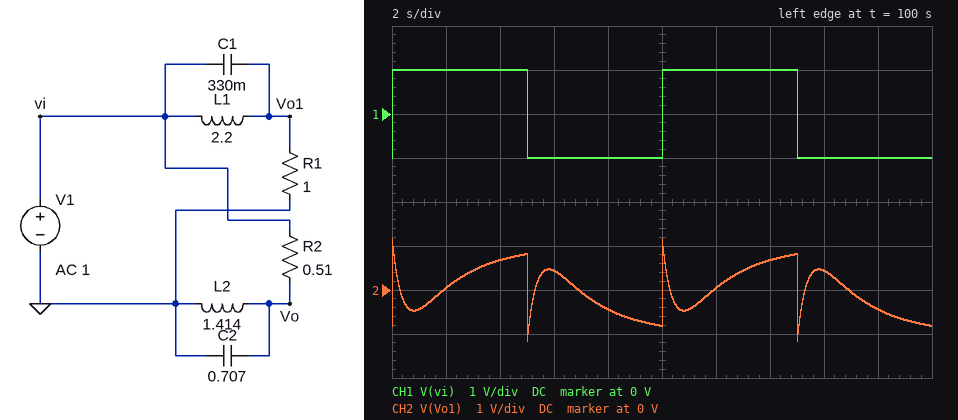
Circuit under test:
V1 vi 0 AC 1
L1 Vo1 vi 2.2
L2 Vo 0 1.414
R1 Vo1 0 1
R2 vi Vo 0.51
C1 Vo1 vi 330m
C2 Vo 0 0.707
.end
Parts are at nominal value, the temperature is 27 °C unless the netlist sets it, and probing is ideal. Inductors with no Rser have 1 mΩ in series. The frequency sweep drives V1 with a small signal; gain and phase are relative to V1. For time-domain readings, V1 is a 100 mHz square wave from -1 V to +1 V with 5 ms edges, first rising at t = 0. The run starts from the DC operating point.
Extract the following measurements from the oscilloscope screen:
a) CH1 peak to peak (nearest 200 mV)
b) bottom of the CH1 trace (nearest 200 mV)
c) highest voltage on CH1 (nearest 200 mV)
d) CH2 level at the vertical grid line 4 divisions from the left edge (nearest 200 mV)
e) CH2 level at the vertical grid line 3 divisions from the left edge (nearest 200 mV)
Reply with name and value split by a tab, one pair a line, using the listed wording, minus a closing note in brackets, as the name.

CH1 peak to peak	2.0 V
bottom of the CH1 trace	-1.0 V
highest voltage on CH1	1.0 V
CH2 level at the vertical grid line 4 divisions from the left edge	-400 mV
CH2 level at the vertical grid line 3 divisions from the left edge	400 mV
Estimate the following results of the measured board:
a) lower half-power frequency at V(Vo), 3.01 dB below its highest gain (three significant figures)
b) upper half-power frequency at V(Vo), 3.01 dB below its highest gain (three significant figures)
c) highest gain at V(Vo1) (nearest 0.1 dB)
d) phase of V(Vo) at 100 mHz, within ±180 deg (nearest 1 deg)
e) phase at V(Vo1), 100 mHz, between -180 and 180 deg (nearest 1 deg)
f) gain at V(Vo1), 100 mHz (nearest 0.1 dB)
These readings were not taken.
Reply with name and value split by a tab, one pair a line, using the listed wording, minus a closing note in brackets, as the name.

lower half-power frequency at V(Vo), 3.01 dB below its highest gain	51.5 mHz
upper half-power frequency at V(Vo), 3.01 dB below its highest gain	493 mHz
highest gain at V(Vo1)	0 dB
phase of V(Vo) at 100 mHz, within ±180 deg	19 deg
phase at V(Vo1), 100 mHz, between -180 and 180 deg	-63 deg
gain at V(Vo1), 100 mHz	-6.8 dB
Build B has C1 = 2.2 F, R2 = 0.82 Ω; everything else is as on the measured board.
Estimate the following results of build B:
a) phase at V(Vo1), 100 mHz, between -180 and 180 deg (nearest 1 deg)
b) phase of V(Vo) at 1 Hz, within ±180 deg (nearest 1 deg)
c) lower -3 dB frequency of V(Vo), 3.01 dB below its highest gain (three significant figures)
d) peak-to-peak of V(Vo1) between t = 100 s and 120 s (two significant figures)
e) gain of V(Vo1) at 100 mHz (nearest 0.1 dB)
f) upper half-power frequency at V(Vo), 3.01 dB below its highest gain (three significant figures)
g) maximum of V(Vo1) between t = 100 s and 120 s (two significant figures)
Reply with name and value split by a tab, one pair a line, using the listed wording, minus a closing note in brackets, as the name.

phase at V(Vo1), 100 mHz, between -180 and 180 deg	57 deg
phase of V(Vo) at 1 Hz, within ±180 deg	-74 deg
lower -3 dB frequency of V(Vo), 3.01 dB below its highest gain	73.0 mHz
peak-to-peak of V(Vo1) between t = 100 s and 120 s	3.6 V
gain of V(Vo1) at 100 mHz	-5.2 dB
upper half-power frequency at V(Vo), 3.01 dB below its highest gain	348 mHz
maximum of V(Vo1) between t = 100 s and 120 s	1.8 V
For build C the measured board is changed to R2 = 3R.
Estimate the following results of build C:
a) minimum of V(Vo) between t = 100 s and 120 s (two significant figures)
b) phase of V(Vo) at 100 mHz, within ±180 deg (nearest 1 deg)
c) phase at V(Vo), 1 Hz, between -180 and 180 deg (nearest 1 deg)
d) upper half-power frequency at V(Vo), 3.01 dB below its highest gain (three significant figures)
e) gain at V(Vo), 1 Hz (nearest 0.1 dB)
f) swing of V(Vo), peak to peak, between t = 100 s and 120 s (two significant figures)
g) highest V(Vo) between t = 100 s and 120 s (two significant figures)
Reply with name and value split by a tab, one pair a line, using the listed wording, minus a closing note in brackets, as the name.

minimum of V(Vo) between t = 100 s and 120 s	-670 mV
phase of V(Vo) at 100 mHz, within ±180 deg	64 deg
phase at V(Vo), 1 Hz, between -180 and 180 deg	-86 deg
upper half-power frequency at V(Vo), 3.01 dB below its highest gain	201 mHz
gain at V(Vo), 1 Hz	-22.3 dB
swing of V(Vo), peak to peak, between t = 100 s and 120 s	1.3 V
highest V(Vo) between t = 100 s and 120 s	670 mV
